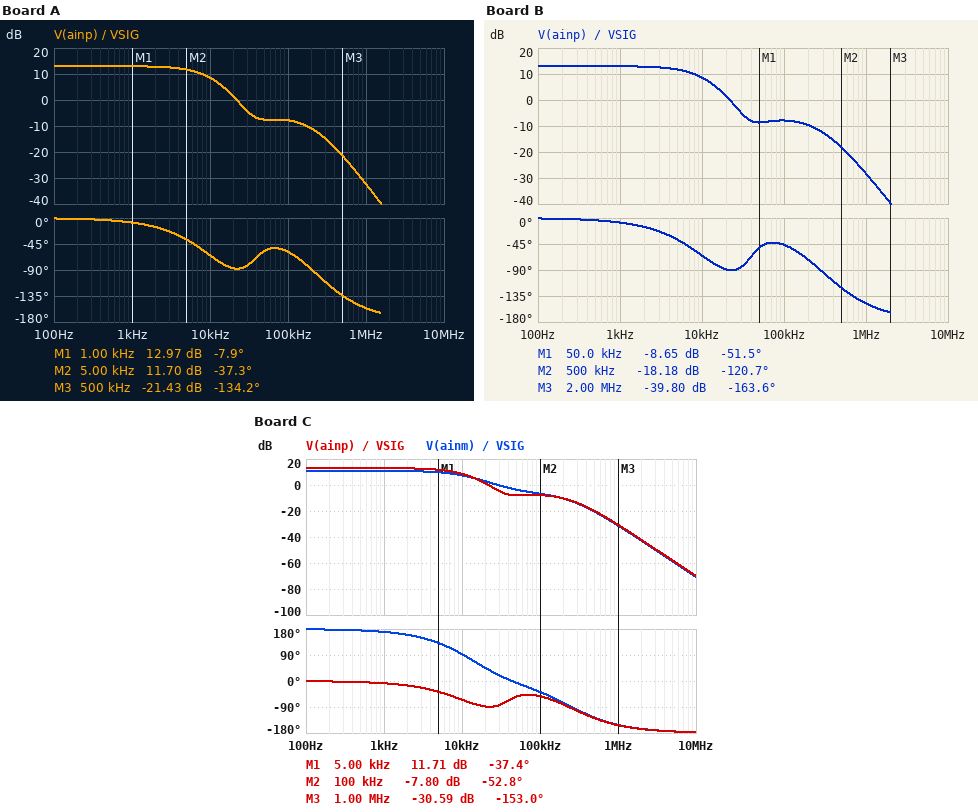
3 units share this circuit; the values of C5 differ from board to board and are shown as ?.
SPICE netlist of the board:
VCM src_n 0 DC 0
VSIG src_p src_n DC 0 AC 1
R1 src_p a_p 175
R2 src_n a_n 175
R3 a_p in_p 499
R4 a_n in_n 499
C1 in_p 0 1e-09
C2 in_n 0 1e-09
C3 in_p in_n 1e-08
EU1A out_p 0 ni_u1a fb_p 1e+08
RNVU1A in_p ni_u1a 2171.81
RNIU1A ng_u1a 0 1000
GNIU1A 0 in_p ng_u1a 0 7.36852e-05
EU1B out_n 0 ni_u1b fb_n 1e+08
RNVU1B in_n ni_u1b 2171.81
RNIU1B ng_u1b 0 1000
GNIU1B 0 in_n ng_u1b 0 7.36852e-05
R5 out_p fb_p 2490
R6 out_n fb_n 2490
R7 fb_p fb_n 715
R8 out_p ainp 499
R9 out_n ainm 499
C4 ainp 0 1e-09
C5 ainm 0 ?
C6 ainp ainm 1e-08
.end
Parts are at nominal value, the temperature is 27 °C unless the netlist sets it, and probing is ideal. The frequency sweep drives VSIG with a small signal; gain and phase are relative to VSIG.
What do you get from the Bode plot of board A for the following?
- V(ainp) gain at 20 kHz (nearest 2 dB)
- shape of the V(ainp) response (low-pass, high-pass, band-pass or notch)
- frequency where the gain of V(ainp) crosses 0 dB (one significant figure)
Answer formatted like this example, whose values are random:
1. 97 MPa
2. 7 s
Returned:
1. 2 dB
2. low-pass
3. 20 kHz
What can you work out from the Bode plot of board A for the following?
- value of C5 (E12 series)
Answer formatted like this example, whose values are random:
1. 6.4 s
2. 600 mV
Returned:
1. 2.2 nF
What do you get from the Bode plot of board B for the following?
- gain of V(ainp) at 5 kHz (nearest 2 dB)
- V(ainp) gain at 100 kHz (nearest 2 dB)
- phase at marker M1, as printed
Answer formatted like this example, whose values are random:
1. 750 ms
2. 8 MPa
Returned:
1. 12 dB
2. -8 dB
3. -51.5 deg
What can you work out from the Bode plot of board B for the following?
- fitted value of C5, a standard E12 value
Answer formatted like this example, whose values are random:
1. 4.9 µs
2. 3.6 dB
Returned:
1. 820 pF
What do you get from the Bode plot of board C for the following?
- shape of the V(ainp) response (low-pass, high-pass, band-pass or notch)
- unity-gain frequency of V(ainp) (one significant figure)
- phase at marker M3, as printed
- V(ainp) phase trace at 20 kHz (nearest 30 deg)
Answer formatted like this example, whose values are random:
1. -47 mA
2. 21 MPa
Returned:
1. low-pass
2. 20 kHz
3. -153.0 deg
4. -90 deg
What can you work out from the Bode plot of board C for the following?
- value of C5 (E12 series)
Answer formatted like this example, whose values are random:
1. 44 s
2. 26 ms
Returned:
1. 1.5 nF
